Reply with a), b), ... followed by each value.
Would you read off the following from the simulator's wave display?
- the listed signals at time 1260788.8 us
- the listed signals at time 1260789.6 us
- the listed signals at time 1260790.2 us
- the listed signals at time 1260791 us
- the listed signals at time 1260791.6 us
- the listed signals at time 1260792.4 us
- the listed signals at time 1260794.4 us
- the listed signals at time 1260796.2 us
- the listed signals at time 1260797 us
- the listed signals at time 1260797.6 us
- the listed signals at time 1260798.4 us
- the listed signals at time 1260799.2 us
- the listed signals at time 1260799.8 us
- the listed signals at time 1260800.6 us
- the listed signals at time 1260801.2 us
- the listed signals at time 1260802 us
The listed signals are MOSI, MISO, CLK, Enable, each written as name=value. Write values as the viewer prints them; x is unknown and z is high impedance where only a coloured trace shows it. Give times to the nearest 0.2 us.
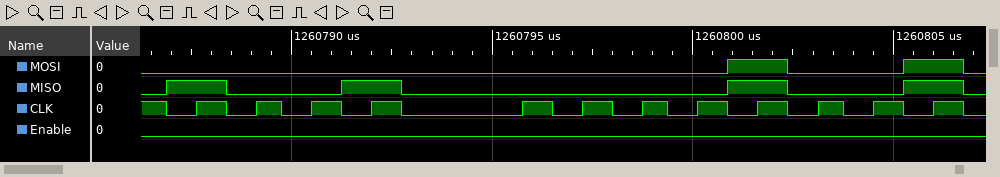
a) MOSI=0, MISO=0, CLK=0, Enable=0
b) MOSI=0, MISO=0, CLK=1, Enable=0
c) MOSI=0, MISO=0, CLK=0, Enable=0
d) MOSI=0, MISO=0, CLK=1, Enable=0
e) MOSI=0, MISO=1, CLK=0, Enable=0
f) MOSI=0, MISO=1, CLK=1, Enable=0
g) MOSI=0, MISO=0, CLK=0, Enable=0
h) MOSI=0, MISO=0, CLK=1, Enable=0
i) MOSI=0, MISO=0, CLK=0, Enable=0
j) MOSI=0, MISO=0, CLK=1, Enable=0
k) MOSI=0, MISO=0, CLK=0, Enable=0
l) MOSI=0, MISO=0, CLK=1, Enable=0
m) MOSI=0, MISO=0, CLK=0, Enable=0
n) MOSI=0, MISO=0, CLK=1, Enable=0
o) MOSI=1, MISO=1, CLK=0, Enable=0
p) MOSI=1, MISO=1, CLK=1, Enable=0
